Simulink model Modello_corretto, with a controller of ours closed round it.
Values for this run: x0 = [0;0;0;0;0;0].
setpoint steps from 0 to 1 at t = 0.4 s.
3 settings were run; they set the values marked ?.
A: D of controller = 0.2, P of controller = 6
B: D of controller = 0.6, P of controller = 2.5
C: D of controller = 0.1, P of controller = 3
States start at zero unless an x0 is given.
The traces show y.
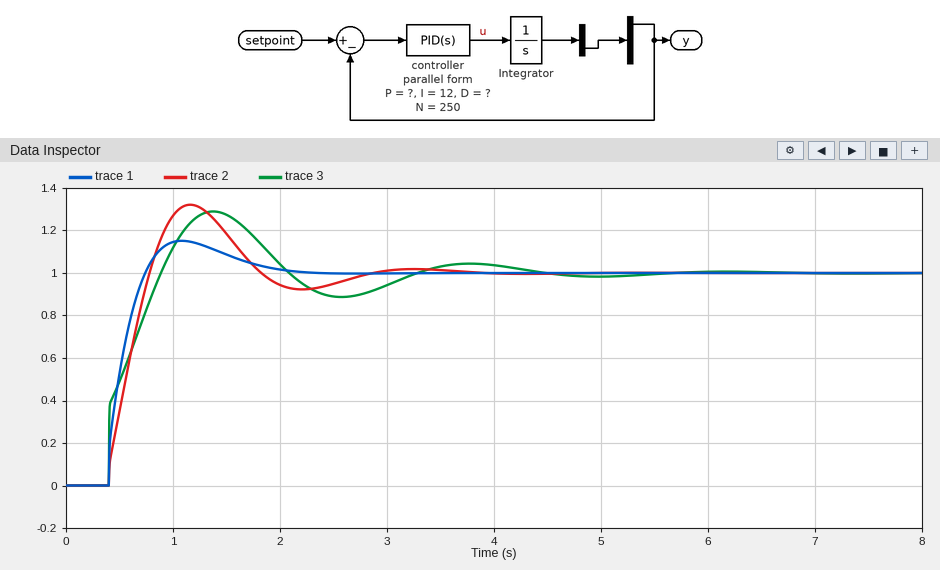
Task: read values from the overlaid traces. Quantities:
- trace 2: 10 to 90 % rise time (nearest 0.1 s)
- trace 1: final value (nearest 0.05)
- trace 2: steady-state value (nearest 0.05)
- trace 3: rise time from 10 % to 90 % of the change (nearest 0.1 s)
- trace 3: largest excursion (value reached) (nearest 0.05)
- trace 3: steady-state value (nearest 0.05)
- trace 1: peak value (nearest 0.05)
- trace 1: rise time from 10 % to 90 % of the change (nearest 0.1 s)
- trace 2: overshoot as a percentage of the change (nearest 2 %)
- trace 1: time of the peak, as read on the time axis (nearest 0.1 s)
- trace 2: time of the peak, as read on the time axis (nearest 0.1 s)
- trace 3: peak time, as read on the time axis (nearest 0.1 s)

0.3 s
1.00
1.00
0.4 s
1.30
1.00
1.15
0.3 s
32 %
1.1 s
1.2 s
1.4 s
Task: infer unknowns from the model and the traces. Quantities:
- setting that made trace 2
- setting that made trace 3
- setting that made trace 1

C
B
A
